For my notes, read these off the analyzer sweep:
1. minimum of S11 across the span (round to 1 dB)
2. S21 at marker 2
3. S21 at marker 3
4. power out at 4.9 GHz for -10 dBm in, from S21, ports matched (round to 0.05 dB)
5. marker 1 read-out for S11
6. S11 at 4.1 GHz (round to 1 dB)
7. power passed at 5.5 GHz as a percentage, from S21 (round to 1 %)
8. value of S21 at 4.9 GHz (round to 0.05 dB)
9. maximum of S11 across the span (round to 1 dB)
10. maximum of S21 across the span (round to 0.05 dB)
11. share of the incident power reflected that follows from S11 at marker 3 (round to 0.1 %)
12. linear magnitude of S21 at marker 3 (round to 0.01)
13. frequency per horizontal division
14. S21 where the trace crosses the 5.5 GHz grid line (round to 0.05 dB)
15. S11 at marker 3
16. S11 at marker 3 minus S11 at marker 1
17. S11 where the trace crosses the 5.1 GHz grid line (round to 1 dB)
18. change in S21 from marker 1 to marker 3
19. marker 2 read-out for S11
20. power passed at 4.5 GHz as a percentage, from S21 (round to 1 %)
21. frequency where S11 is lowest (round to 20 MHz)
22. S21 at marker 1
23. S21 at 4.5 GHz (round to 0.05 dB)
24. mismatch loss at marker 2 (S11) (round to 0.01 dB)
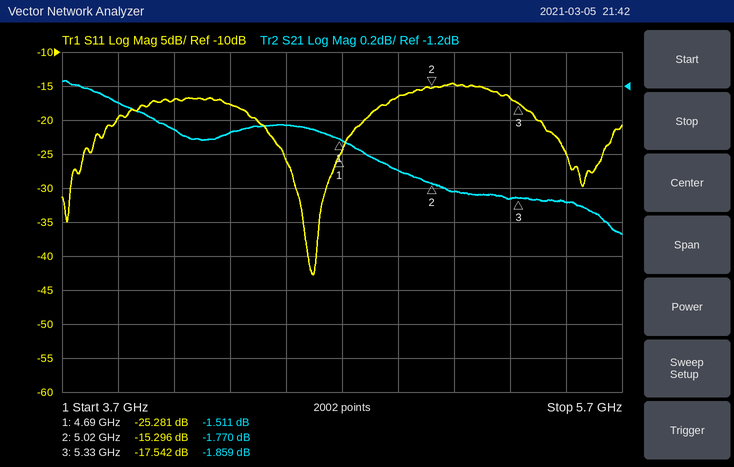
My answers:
-43 dB
-1.770 dB
-1.859 dB
-11.70 dBm
-25.281 dB
-17 dB
65 %
-1.70 dB
-15 dB
-1.15 dB
1.8 %
0.81
200 MHz
-1.90 dB
-17.542 dB
7.739 dB
-15 dB
-0.348 dB
-15.296 dB
72 %
4.60 GHz
-1.511 dB
-1.45 dB
0.13 dB
